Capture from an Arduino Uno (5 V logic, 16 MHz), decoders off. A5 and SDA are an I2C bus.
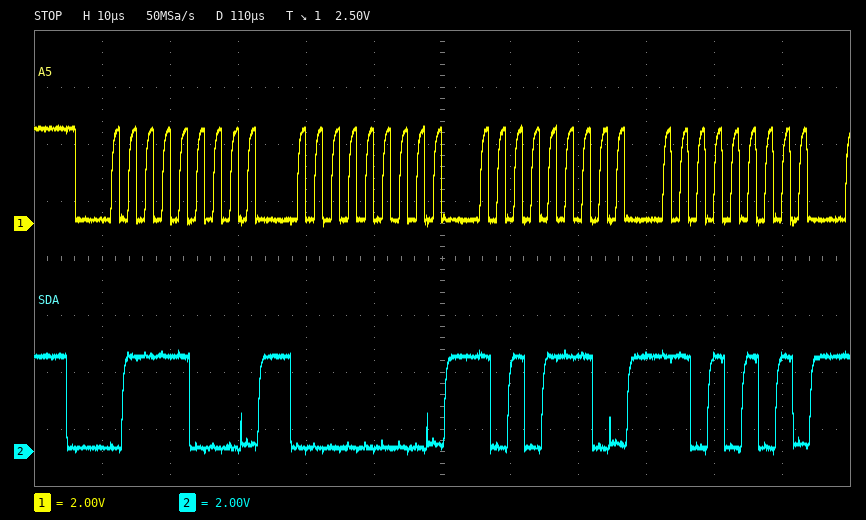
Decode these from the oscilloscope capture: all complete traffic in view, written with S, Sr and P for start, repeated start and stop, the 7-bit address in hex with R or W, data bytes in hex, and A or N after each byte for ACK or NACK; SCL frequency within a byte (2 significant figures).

S 3CW A 00 A AE A D5 A
400 kHz
